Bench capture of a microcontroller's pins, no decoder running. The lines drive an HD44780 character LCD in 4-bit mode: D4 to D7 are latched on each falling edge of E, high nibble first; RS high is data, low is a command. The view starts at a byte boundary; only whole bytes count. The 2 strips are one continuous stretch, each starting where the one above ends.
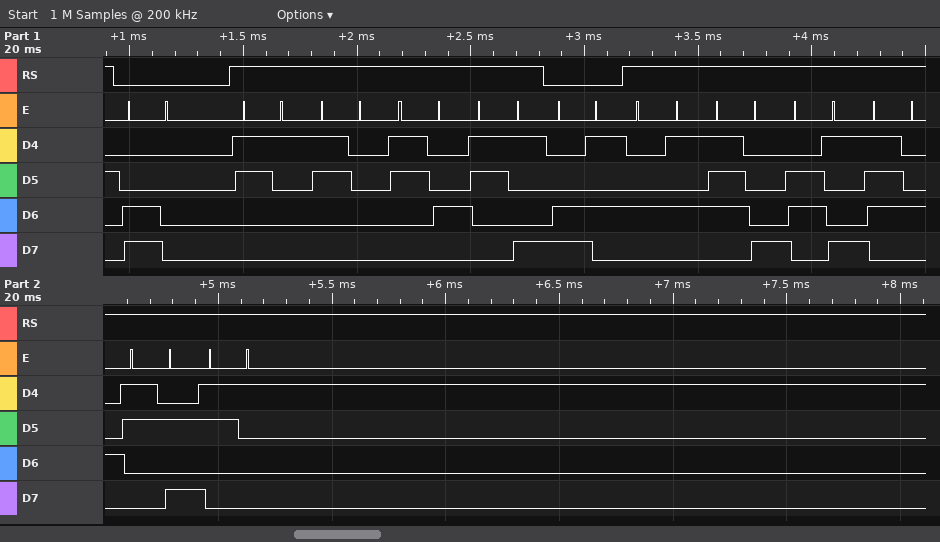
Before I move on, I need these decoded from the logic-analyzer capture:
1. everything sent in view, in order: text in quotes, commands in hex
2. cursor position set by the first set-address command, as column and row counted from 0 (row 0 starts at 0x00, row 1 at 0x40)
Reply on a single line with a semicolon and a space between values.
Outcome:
0xC0 "1049" 0xC5 "Exit:1"; column 0, row 1
